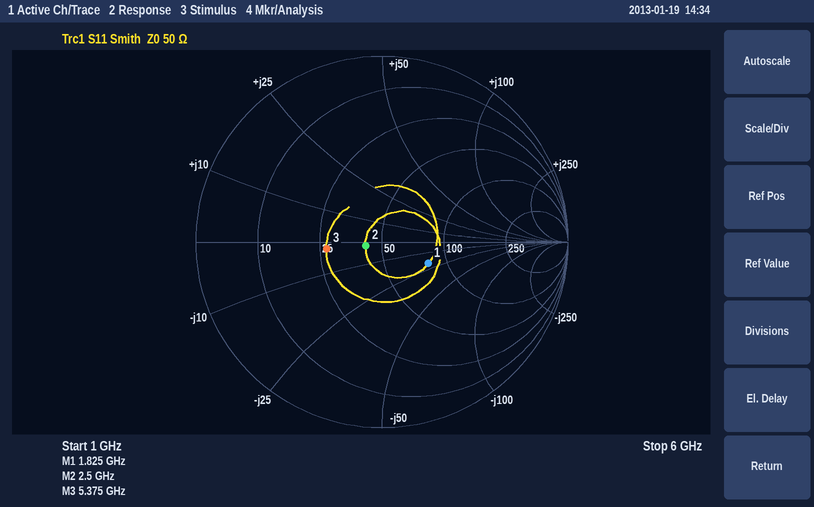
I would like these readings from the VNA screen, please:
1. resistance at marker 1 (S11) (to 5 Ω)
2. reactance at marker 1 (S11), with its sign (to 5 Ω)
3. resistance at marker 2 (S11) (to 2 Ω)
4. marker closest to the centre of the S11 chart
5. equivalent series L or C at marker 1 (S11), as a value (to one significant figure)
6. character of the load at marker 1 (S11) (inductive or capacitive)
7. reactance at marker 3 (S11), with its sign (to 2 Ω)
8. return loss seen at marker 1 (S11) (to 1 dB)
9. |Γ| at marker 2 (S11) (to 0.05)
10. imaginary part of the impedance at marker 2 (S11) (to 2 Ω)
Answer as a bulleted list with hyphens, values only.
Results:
- 80 Ω
- -20 Ω
- 42 Ω
- marker 2
- 4 pF
- capacitive
- -2 Ω
- 11 dB
- 0.10
- -2 Ω
